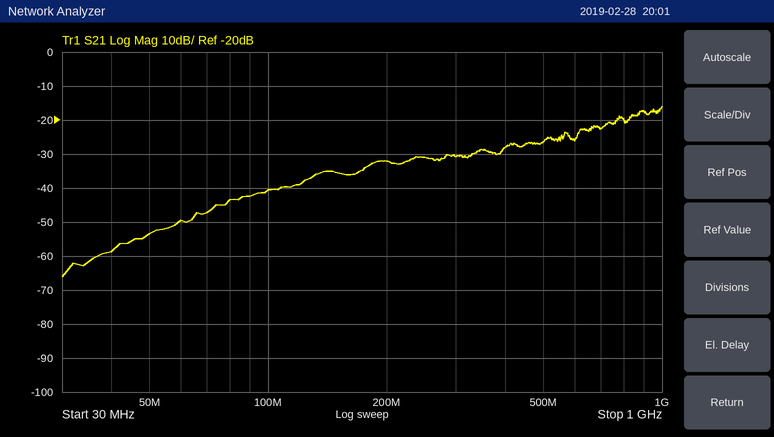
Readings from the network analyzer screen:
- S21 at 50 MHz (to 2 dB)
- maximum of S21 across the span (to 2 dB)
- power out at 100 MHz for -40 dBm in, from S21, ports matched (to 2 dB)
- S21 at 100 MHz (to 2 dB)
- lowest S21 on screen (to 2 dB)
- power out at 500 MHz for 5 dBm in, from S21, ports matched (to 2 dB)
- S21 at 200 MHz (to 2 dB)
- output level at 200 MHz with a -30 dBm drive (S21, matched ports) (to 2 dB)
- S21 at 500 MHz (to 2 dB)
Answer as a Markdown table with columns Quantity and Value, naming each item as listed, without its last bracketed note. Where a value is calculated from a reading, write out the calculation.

| Quantity | Value |
|---|---|
| S21 at 50 MHz | -54 dB |
| maximum of S21 across the span | -16 dB |
| power out at 100 MHz for -40 dBm in, from S21, ports matched | -40 dBm + (-40 dB) = -80 dBm |
| S21 at 100 MHz | -40 dB |
| lowest S21 on screen | -66 dB |
| power out at 500 MHz for 5 dBm in, from S21, ports matched | 5 dBm + (-26 dB) = -22 dBm |
| S21 at 200 MHz | -32 dB |
| output level at 200 MHz with a -30 dBm drive (S21, matched ports) | -30 dBm + (-32 dB) = -62 dBm |
| S21 at 500 MHz | -26 dB |
